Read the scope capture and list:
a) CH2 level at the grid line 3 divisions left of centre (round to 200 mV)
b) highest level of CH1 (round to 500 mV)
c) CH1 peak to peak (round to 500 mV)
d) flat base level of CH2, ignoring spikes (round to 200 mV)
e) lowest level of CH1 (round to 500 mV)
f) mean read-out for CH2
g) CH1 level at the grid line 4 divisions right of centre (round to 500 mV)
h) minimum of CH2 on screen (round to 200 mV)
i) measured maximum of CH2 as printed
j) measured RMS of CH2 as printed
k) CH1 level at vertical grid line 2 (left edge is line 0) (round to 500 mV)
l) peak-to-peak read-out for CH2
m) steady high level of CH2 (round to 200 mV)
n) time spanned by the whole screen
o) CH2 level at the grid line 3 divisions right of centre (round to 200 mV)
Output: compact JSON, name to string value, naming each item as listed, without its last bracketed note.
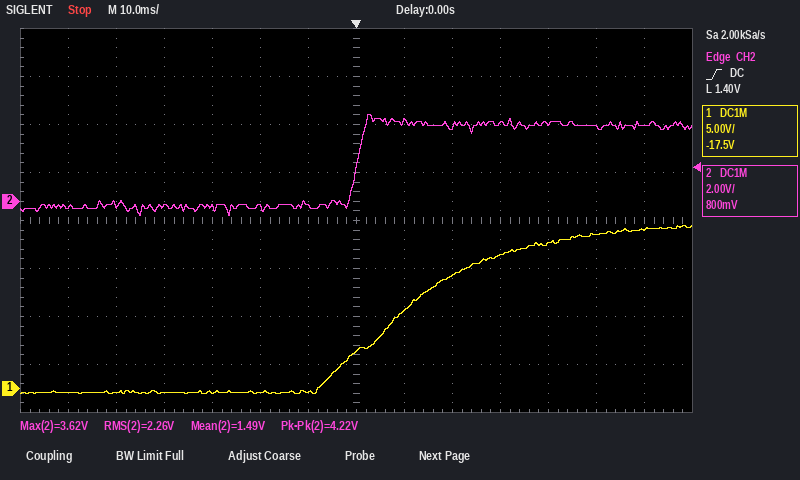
{"CH2 level at the grid line 3 divisions left of centre": "-200 mV", "highest level of CH1": "17.0 V", "CH1 peak to peak": "17.5 V", "flat base level of CH2, ignoring spikes": "-200 mV", "lowest level of CH1": "-500 mV", "mean read-out for CH2": "1.49 V", "CH1 level at the grid line 4 divisions right of centre": "15.0 V", "minimum of CH2 on screen": "-600 mV", "measured maximum of CH2 as printed": "3.62 V", "measured RMS of CH2 as printed": "2.26 V", "CH1 level at vertical grid line 2 (left edge is line 0)": "-500 mV", "peak-to-peak read-out for CH2": "4.22 V", "steady high level of CH2": "3.2 V", "time spanned by the whole screen": "140 ms", "CH2 level at the grid line 3 divisions right of centre": "3.2 V"}
